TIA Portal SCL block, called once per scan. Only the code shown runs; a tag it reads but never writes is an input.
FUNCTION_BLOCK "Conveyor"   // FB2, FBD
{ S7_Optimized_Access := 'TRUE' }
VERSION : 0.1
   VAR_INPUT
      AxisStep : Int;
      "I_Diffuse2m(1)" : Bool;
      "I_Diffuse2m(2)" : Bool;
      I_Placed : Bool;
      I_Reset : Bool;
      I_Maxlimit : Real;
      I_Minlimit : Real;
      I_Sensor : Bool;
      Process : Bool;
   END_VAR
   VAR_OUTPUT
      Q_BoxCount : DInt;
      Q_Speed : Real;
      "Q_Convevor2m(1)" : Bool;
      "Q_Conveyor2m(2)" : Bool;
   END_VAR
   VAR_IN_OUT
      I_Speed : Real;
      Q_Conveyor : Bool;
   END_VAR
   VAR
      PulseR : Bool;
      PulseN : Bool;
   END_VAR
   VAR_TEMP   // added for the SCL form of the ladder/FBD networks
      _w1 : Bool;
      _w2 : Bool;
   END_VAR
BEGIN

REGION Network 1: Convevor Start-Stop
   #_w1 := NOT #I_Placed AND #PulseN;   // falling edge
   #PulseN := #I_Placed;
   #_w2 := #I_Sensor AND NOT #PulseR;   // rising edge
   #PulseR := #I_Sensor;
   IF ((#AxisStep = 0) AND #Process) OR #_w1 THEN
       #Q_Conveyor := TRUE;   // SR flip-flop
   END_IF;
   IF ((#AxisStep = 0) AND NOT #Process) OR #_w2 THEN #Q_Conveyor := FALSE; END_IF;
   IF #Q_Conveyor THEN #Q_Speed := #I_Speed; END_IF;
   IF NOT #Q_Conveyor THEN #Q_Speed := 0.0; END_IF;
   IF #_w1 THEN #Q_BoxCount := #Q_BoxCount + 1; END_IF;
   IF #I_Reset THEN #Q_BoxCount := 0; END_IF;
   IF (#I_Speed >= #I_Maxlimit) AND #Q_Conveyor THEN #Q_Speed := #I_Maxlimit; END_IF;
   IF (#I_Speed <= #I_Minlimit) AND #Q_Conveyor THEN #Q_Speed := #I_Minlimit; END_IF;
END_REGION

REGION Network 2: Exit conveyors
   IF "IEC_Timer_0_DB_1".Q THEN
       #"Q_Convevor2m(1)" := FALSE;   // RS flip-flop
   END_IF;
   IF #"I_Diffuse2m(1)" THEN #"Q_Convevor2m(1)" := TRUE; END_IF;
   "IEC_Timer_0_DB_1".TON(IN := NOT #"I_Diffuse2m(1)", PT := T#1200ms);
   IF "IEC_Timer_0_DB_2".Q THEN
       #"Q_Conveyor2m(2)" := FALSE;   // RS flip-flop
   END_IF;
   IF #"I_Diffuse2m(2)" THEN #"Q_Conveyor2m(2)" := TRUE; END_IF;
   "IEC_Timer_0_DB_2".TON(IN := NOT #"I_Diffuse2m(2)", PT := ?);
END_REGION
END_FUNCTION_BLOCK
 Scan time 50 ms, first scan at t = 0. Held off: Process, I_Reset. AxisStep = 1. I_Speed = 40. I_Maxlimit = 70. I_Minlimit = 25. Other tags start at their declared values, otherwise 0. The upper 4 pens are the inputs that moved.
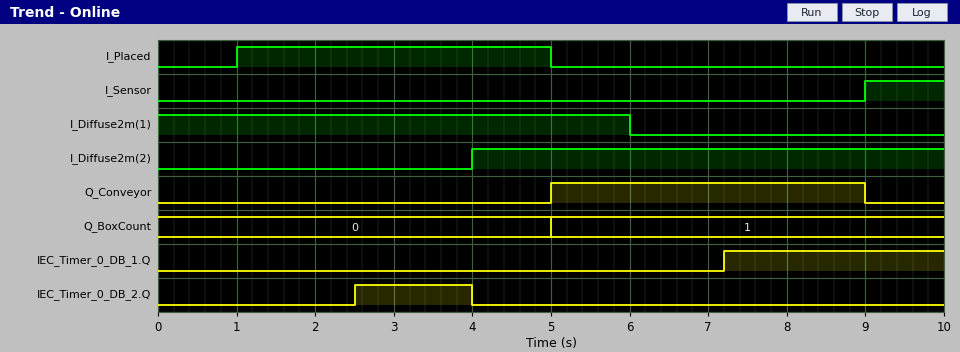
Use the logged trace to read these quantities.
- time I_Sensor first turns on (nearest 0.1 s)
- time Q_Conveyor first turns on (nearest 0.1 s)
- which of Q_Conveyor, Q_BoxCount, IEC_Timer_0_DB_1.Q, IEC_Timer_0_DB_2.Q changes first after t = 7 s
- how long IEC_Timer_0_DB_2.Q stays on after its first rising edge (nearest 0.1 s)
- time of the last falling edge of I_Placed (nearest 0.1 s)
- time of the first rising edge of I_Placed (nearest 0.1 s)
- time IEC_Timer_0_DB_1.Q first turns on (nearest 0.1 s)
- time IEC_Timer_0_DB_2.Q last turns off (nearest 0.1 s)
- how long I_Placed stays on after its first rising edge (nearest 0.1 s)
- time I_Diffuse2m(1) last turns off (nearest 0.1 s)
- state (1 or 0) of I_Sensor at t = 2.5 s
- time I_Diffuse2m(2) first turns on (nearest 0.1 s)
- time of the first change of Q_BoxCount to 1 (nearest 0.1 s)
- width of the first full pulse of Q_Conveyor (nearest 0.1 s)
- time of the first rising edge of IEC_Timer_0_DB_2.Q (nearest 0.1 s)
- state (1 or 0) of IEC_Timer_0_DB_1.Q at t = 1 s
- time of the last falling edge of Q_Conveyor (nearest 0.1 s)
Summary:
9.0 s
5.0 s
IEC_Timer_0_DB_1.Q
1.5 s
5.0 s
1.0 s
7.2 s
4.0 s
4.0 s
6.0 s
0
4.0 s
5.0 s
4.0 s
2.5 s
0
9.0 s
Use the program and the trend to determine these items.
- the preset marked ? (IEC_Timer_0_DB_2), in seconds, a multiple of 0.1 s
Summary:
2.5 s
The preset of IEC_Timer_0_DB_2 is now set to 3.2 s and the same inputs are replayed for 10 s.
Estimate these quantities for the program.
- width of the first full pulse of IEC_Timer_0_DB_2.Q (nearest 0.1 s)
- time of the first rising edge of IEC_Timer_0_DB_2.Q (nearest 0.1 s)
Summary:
0.8 s
3.2 s
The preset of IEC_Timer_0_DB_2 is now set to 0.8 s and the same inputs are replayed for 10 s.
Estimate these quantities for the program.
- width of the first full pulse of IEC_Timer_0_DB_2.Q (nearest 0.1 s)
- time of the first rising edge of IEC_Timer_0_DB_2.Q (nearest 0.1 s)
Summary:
3.2 s
0.8 s
